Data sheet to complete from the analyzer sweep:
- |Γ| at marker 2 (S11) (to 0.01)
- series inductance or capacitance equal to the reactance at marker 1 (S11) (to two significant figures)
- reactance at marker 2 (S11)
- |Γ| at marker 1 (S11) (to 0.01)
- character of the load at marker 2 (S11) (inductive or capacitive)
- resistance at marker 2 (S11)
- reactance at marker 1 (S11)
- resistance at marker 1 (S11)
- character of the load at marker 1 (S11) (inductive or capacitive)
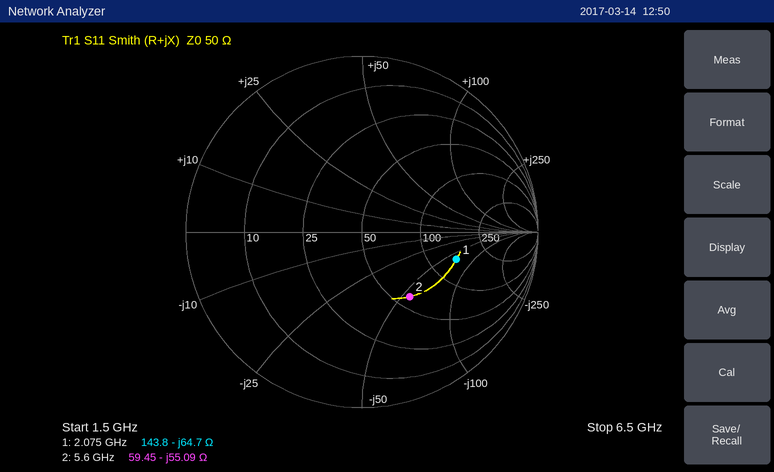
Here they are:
0.46
1.2 pF
-55.09 Ω
0.56
capacitive
59.45 Ω
-64.7 Ω
143.8 Ω
capacitive
